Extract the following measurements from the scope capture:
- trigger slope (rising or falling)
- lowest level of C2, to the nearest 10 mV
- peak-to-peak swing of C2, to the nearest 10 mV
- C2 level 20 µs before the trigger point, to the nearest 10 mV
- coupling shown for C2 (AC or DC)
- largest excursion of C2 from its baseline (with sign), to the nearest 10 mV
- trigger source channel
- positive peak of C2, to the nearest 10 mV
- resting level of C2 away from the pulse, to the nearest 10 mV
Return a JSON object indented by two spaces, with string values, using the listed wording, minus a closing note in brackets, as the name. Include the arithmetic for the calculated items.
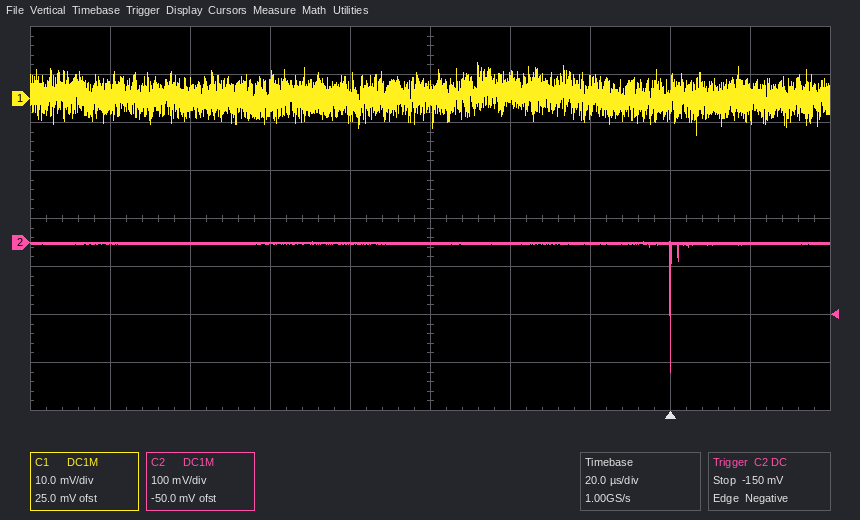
{
  "trigger slope": "falling",
  "lowest level of C2, to the nearest 10 mV": "-270 mV",
  "peak-to-peak swing of C2, to the nearest 10 mV": "0 mV − (-270 mV) = 270 mV",
  "C2 level 20 µs before the trigger point, to the nearest 10 mV": "0 mV",
  "coupling shown for C2": "DC",
  "largest excursion of C2 from its baseline (with sign), to the nearest 10 mV": "-270 mV − (0 mV) = -270 mV",
  "trigger source channel": "C2",
  "positive peak of C2, to the nearest 10 mV": "0 mV",
  "resting level of C2 away from the pulse, to the nearest 10 mV": "0 mV"
}
